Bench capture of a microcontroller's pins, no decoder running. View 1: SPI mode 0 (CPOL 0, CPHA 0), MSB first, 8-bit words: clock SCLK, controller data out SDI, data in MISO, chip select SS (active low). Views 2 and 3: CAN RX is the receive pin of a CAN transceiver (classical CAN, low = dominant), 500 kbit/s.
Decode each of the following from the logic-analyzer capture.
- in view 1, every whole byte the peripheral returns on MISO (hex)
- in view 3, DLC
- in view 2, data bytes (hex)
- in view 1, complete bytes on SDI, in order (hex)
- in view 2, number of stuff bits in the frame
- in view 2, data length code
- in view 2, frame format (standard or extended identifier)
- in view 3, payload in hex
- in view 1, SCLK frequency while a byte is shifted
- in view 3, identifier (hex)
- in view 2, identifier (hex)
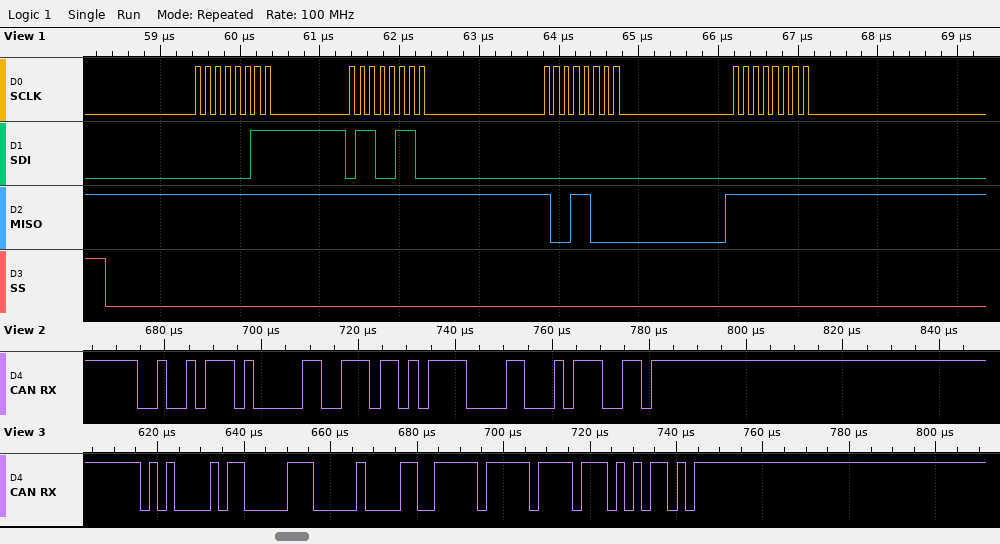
FF FF 98 FF
3
76 BC
03 66 00 00
1
2
standard
00 67 FF
8 MHz
0x50B
0x25D
